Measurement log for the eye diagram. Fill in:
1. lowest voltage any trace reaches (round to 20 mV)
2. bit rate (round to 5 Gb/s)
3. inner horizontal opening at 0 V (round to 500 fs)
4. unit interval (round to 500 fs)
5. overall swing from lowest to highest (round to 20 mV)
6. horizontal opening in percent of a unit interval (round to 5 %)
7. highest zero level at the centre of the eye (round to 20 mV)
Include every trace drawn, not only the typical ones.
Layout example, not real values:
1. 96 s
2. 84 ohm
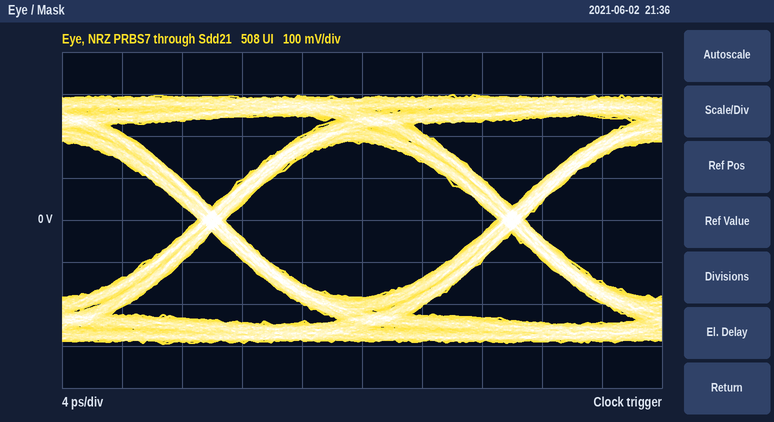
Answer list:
1. -300 mV
2. 50 Gb/s
3. 18.0 ps
4. 20.0 ps
5. 600 mV
6. 90 %
7. -180 mV
